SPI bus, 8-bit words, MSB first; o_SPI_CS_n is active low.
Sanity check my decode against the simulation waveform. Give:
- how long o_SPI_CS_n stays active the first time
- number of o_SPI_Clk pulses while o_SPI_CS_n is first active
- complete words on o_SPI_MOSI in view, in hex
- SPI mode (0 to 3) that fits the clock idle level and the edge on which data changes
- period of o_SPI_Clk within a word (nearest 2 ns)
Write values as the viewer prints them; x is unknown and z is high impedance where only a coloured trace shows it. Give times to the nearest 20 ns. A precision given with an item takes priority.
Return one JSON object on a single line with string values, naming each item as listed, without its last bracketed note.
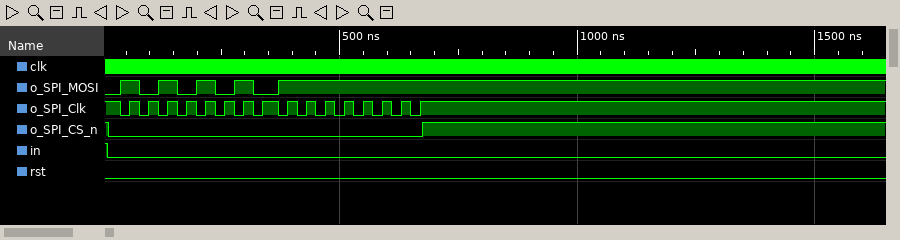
{"how long o_SPI_CS_n stays active the first time": "660 ns", "number of o_SPI_Clk pulses while o_SPI_CS_n is first active": "16", "complete words on o_SPI_MOSI in view, in hex": "AA, FF", "SPI mode (0 to 3) that fits the clock idle level and the edge on which data changes": "3", "period of o_SPI_Clk within a word": "40 ns"}
